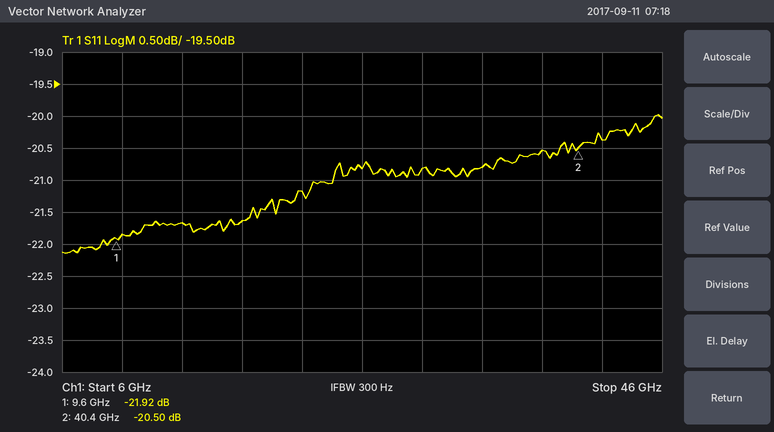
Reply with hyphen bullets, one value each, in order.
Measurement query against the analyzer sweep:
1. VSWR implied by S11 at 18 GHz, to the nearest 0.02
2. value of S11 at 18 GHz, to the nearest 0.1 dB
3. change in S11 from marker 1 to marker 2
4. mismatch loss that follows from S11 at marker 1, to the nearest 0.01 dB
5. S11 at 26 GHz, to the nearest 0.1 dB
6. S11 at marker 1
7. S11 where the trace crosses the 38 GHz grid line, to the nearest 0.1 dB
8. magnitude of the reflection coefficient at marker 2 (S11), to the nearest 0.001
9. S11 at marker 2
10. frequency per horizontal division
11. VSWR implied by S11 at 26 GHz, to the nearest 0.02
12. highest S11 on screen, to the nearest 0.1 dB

- 1.18
- -21.6 dB
- 1.42 dB
- 0.03 dB
- -20.8 dB
- -21.92 dB
- -20.5 dB
- 0.094
- -20.50 dB
- 4 GHz
- 1.20
- -20.0 dB
